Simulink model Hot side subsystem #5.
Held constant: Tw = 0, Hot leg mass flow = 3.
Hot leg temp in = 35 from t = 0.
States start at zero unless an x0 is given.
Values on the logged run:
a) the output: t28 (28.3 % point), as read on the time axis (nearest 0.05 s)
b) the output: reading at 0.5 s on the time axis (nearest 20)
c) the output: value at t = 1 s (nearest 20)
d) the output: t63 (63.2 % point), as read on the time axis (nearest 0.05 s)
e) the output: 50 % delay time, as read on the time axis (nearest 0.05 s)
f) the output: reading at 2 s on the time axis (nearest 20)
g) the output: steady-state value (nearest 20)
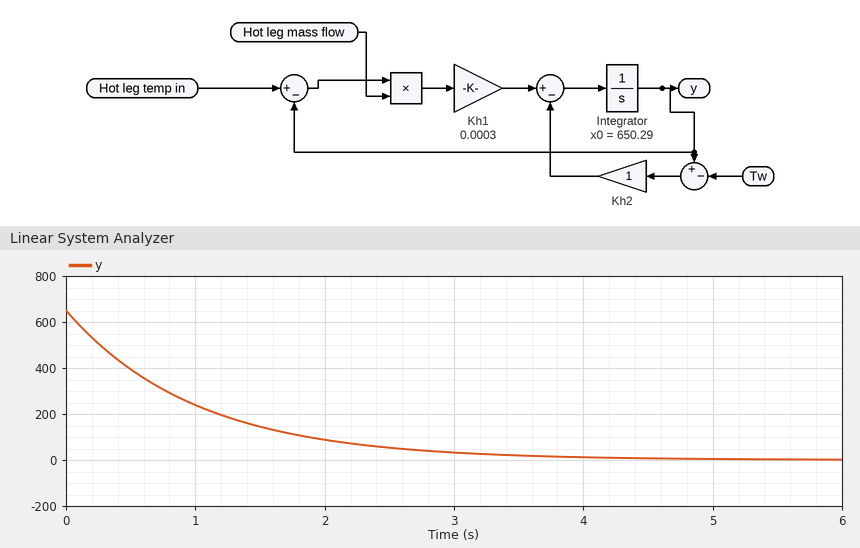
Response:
0.35 s
400
240
1.00 s
0.70 s
80
0
